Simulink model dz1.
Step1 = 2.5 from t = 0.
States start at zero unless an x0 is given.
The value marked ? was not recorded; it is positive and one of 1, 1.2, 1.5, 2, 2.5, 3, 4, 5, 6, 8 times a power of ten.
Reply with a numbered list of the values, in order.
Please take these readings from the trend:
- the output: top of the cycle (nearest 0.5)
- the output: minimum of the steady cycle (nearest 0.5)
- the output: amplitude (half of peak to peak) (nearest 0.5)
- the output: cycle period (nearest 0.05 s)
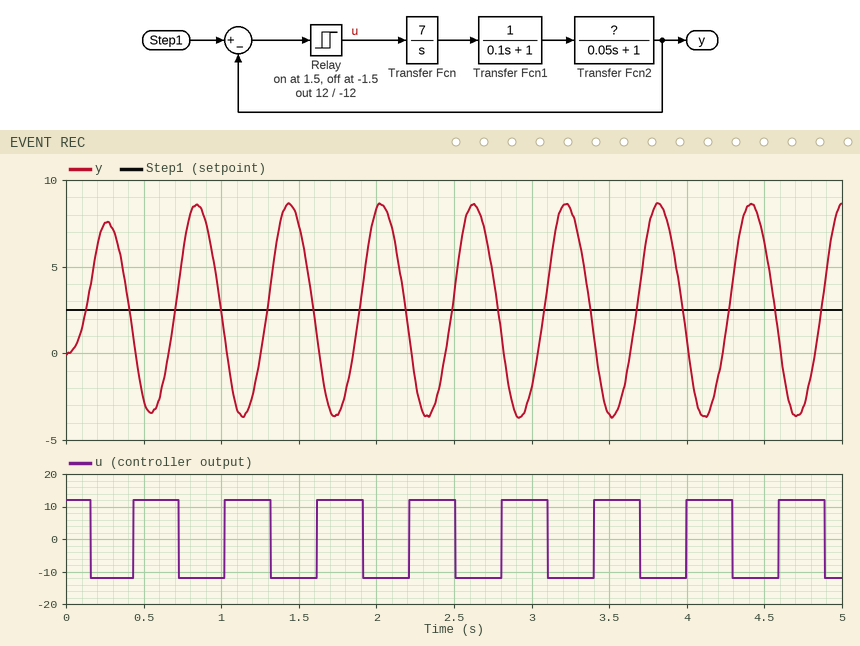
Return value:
1. 8.5
2. -3.5
3. 6.0
4. 0.60 s
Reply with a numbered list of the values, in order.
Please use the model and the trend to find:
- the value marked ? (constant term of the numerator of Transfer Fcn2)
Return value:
1. 1
